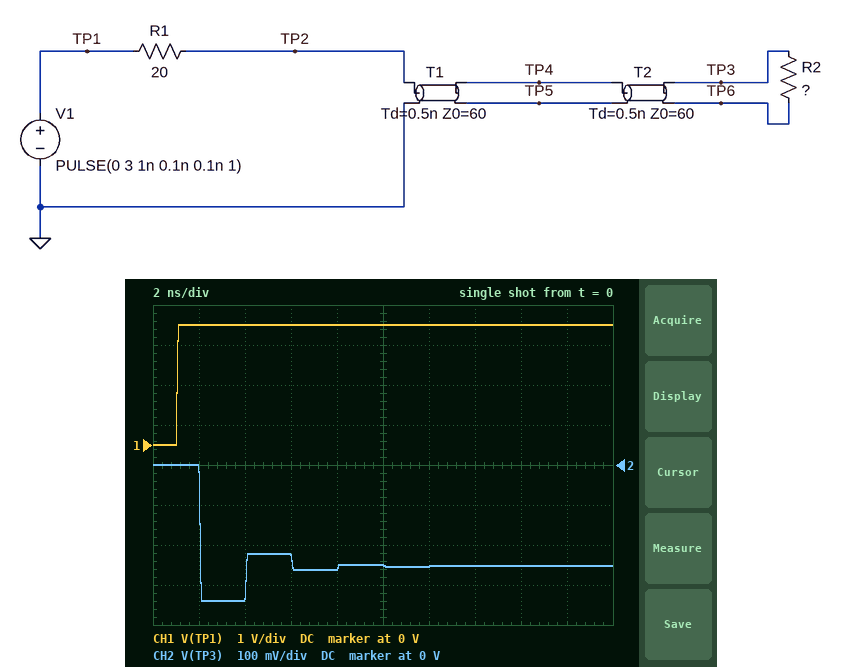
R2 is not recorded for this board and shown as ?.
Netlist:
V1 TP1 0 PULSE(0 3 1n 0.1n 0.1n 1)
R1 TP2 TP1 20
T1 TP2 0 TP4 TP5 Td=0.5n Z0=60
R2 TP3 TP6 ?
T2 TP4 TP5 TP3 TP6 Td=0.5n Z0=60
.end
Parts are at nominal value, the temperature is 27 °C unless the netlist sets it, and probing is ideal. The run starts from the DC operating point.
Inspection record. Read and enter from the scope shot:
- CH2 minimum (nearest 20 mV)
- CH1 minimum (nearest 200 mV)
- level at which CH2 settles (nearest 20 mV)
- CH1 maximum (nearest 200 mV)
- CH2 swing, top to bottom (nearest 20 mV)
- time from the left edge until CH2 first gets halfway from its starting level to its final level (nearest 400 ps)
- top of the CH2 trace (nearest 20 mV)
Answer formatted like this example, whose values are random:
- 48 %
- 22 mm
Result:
- -340 mV
- 0 V
- -260 mV
- 3.0 V
- 340 mV
- 2.0 ns
- 0 V
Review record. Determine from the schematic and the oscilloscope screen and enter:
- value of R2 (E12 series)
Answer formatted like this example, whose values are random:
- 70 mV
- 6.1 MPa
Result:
- 330 Ω
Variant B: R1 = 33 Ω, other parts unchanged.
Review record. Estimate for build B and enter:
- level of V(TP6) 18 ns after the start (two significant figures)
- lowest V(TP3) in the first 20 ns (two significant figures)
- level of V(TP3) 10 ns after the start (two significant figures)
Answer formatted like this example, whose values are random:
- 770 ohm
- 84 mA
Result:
- -3.0 V
- -290 mV
- -240 mV
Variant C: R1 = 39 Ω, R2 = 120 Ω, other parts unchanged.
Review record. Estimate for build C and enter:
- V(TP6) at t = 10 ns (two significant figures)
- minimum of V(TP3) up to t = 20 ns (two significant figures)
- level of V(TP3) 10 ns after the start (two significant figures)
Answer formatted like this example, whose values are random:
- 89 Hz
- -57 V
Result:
- -2.8 V
- -600 mV
- -560 mV
